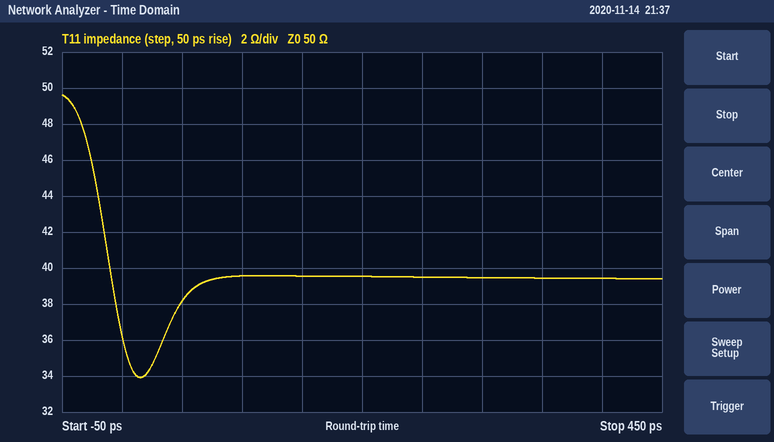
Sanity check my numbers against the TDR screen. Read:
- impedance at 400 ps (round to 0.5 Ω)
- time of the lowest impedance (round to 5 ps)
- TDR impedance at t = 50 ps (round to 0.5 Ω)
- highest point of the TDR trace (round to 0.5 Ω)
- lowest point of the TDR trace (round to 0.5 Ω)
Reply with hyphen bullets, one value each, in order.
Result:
- 39.5 Ω
- 15 ps
- 38.0 Ω
- 49.5 Ω
- 34.0 Ω
